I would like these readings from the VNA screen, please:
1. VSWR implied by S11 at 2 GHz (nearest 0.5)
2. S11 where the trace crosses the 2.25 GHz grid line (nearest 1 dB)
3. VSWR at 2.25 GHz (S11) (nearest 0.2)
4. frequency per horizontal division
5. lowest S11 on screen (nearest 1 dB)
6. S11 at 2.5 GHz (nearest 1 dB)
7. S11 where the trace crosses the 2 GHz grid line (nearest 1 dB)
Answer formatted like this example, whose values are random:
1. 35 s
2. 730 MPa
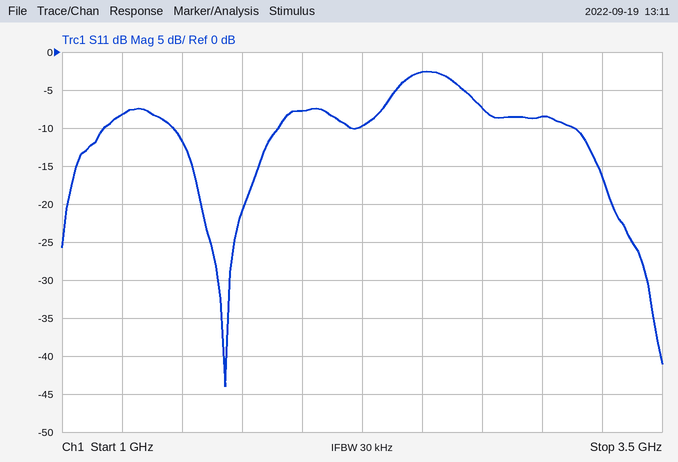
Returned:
1. 2.5
2. -10 dB
3. 2.0
4. 250 MHz
5. -44 dB
6. -3 dB
7. -8 dB
